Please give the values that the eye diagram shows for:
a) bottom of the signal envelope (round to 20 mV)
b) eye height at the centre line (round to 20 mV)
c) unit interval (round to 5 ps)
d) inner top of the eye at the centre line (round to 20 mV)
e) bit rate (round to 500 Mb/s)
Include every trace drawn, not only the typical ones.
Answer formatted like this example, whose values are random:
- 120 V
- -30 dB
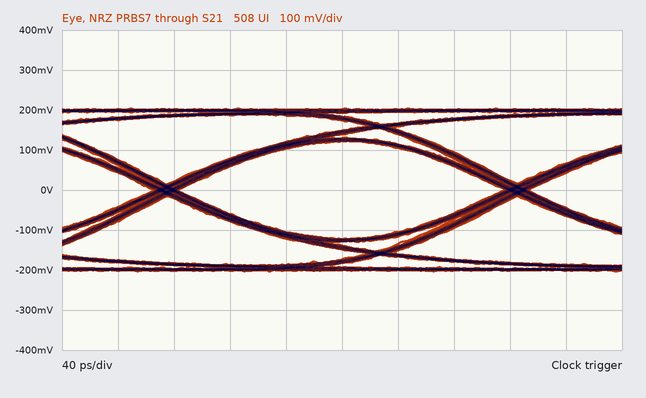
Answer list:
- -200 mV
- 240 mV
- 250 ps
- 120 mV
- 4.0 Gb/s
